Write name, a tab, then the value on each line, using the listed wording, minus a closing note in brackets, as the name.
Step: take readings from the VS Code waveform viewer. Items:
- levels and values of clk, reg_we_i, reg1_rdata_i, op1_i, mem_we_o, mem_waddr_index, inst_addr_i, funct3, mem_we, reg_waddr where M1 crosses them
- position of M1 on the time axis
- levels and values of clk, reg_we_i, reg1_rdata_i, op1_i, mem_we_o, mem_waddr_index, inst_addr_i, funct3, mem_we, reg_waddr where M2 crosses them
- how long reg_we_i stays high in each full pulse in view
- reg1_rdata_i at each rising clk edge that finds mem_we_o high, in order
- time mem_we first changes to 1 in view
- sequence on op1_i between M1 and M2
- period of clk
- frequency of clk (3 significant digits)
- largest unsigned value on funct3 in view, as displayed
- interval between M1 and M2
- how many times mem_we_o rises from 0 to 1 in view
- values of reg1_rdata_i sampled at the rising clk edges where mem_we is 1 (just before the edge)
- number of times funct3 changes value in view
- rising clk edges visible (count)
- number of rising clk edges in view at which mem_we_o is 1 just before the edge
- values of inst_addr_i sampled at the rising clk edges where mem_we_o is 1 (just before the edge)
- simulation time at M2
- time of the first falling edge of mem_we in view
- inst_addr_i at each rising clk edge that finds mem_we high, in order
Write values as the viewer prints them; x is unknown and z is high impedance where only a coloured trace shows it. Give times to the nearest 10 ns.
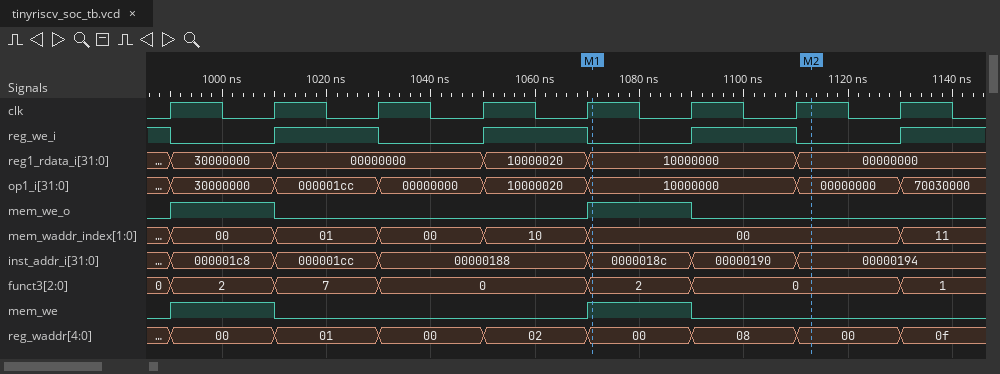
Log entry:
levels and values of clk, reg_we_i, reg1_rdata_i, op1_i, mem_we_o, mem_waddr_index, inst_addr_i, funct3, mem_we, reg_waddr where M1 crosses them	clk=1, reg_we_i=0, reg1_rdata_i=10000000, op1_i=10000000, mem_we_o=1, mem_waddr_index=00, inst_addr_i=0000018c, funct3=2, mem_we=1, reg_waddr=00
position of M1 on the time axis	1070 ns
levels and values of clk, reg_we_i, reg1_rdata_i, op1_i, mem_we_o, mem_waddr_index, inst_addr_i, funct3, mem_we, reg_waddr where M2 crosses them	clk=1, reg_we_i=0, reg1_rdata_i=00000000, op1_i=00000000, mem_we_o=0, mem_waddr_index=00, inst_addr_i=00000194, funct3=0, mem_we=0, reg_waddr=00
how long reg_we_i stays high in each full pulse in view	20 ns, 20 ns, 20 ns
reg1_rdata_i at each rising clk edge that finds mem_we_o high, in order	30000000, 10000000
time mem_we first changes to 1 in view	990 ns
sequence on op1_i between M1 and M2	10000000, 00000000
period of clk	20 ns
frequency of clk	50.0 MHz
largest unsigned value on funct3 in view, as displayed	7
interval between M1 and M2	40 ns
how many times mem_we_o rises from 0 to 1 in view	2
values of reg1_rdata_i sampled at the rising clk edges where mem_we is 1	30000000, 10000000
number of times funct3 changes value in view	6
rising clk edges visible	8
number of rising clk edges in view at which mem_we_o is 1 just before the edge	2
values of inst_addr_i sampled at the rising clk edges where mem_we_o is 1	000001c8, 0000018c
simulation time at M2	1110 ns
time of the first falling edge of mem_we in view	1010 ns
inst_addr_i at each rising clk edge that finds mem_we high, in order	000001c8, 0000018c
